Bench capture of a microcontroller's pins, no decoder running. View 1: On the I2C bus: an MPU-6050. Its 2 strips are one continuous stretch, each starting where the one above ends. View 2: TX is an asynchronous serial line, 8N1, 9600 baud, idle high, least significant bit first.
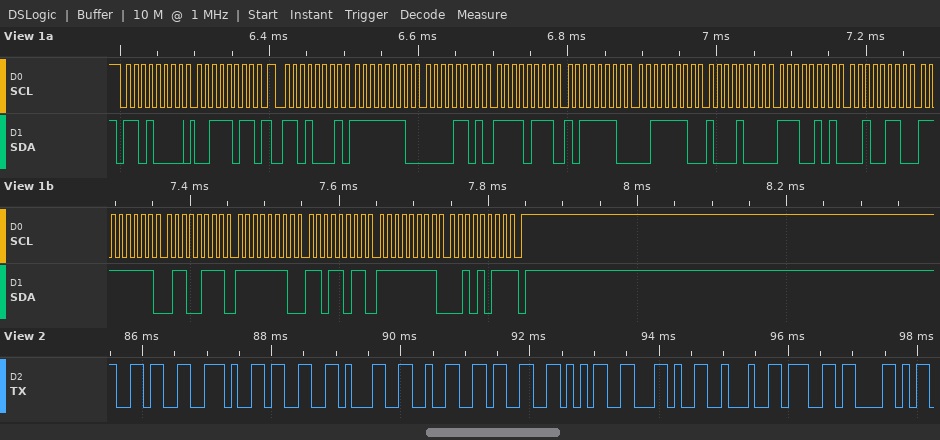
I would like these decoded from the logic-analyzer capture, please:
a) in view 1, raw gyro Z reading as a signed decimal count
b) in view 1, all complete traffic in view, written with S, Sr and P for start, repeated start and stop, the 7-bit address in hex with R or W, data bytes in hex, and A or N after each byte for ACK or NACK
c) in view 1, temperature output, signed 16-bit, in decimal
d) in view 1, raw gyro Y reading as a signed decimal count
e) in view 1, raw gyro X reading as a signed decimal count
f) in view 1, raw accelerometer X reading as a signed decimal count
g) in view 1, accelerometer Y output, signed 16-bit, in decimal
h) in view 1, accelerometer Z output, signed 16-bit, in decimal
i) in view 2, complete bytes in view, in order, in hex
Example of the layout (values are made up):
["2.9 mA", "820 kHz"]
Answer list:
["-213", "S 68W A 3B A Sr 68R A FE A 0D A F7 A BE A 3E A 88 A E5 A 26 A FF A 67 A FE A DB A FF A 2B N P", "-6874", "-293", "-153", "-499", "-2114", "16008", "36 2E 33 31 32 33 35 2C 22 67 58"]
